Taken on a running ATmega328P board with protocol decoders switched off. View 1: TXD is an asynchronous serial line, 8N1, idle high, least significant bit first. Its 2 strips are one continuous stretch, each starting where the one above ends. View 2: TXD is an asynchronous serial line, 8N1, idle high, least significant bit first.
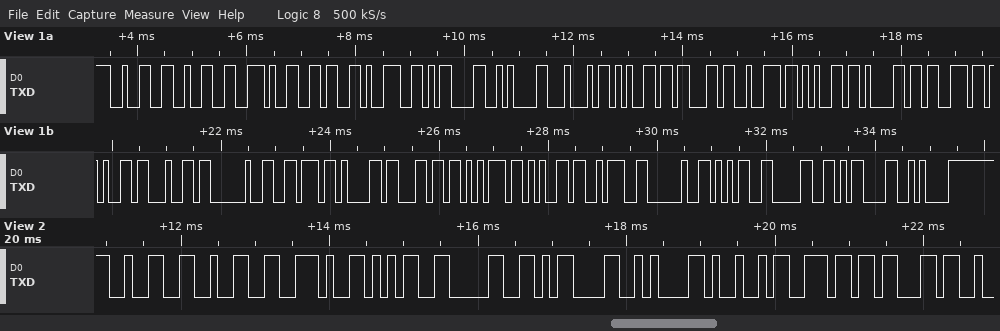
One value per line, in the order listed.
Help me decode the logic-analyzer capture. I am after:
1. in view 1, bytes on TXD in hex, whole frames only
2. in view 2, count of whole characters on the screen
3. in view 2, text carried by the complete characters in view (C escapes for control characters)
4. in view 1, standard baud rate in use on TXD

32 32 2E 36 39 0D 0A 44 65 63 72 65 61 73 65 64 20 76 61 6C 75 65 3A 20 35 30 0D 0A
10
"22.50\r\nInc"
9600 baud
